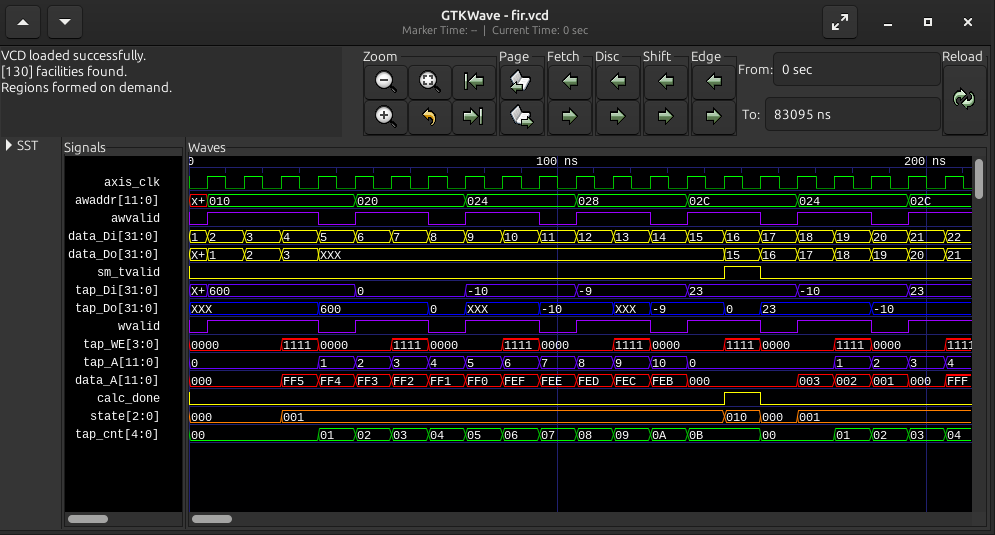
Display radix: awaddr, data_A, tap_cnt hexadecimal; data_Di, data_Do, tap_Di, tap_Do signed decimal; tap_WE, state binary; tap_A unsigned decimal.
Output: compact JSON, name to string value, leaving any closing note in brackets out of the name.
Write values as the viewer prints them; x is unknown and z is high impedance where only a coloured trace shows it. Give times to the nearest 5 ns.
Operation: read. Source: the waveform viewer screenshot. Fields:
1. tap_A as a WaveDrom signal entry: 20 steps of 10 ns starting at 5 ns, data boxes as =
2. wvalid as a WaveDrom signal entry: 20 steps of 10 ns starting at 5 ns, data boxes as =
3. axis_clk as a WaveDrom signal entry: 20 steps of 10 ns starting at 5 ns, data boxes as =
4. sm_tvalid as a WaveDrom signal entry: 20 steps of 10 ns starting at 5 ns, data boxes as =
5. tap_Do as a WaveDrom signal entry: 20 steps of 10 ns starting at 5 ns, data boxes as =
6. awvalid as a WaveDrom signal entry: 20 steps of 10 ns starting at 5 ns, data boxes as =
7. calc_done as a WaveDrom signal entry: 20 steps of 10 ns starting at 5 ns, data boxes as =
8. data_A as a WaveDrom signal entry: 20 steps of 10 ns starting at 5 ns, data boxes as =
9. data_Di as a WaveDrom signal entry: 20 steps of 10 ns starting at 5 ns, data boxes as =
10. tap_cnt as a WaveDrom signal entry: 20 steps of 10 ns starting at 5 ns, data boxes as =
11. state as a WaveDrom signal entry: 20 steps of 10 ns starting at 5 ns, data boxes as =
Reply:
{"tap_A as a WaveDrom signal entry: 20 steps of 10 ns starting at 5 ns, data boxes as =": "{name: 'tap_A', wave: '=..===========...===', data: '0 1 2 3 4 5 6 7 8 9 10 0 1 2 3'}", "wvalid as a WaveDrom signal entry: 20 steps of 10 ns starting at 5 ns, data boxes as =": "{name: 'wvalid', wave: '1..01.01.01.01.01.01'}", "axis_clk as a WaveDrom signal entry: 20 steps of 10 ns starting at 5 ns, data boxes as =": "{name: 'axis_clk', wave: 'p...................'}", "sm_tvalid as a WaveDrom signal entry: 20 steps of 10 ns starting at 5 ns, data boxes as =": "{name: 'sm_tvalid', wave: '0.............10....'}", "tap_Do as a WaveDrom signal entry: 20 steps of 10 ns starting at 5 ns, data boxes as =": "{name: 'tap_Do', wave: 'x..=..=x.=.x=.==..=.', data: '600 0 -10 -9 0 23 -10'}", "awvalid as a WaveDrom signal entry: 20 steps of 10 ns starting at 5 ns, data boxes as =": "{name: 'awvalid', wave: '1..01.01.01.01.01.01'}", "calc_done as a WaveDrom signal entry: 20 steps of 10 ns starting at 5 ns, data boxes as =": "{name: 'calc_done', wave: '0.............10....'}", "data_A as a WaveDrom signal entry: 20 steps of 10 ns starting at 5 ns, data boxes as =": "{name: 'data_A', wave: '=.============..====', data: '000 FF5 FF4 FF3 FF2 FF1 FF0 FEF FEE FED FEC FEB 000 003 002 001 000'}", "data_Di as a WaveDrom signal entry: 20 steps of 10 ns starting at 5 ns, data boxes as =": "{name: 'data_Di', wave: '====================', data: '2 3 4 5 6 7 8 9 10 11 12 13 14 15 16 17 18 19 20 21'}", "tap_cnt as a WaveDrom signal entry: 20 steps of 10 ns starting at 5 ns, data boxes as =": "{name: 'tap_cnt', wave: '=..===========.=.===', data: '00 01 02 03 04 05 06 07 08 09 0A 0B 00 01 02 03'}", "state as a WaveDrom signal entry: 20 steps of 10 ns starting at 5 ns, data boxes as =": "{name: 'state', wave: '=.=...........===...', data: '000 001 010 000 001'}"}
